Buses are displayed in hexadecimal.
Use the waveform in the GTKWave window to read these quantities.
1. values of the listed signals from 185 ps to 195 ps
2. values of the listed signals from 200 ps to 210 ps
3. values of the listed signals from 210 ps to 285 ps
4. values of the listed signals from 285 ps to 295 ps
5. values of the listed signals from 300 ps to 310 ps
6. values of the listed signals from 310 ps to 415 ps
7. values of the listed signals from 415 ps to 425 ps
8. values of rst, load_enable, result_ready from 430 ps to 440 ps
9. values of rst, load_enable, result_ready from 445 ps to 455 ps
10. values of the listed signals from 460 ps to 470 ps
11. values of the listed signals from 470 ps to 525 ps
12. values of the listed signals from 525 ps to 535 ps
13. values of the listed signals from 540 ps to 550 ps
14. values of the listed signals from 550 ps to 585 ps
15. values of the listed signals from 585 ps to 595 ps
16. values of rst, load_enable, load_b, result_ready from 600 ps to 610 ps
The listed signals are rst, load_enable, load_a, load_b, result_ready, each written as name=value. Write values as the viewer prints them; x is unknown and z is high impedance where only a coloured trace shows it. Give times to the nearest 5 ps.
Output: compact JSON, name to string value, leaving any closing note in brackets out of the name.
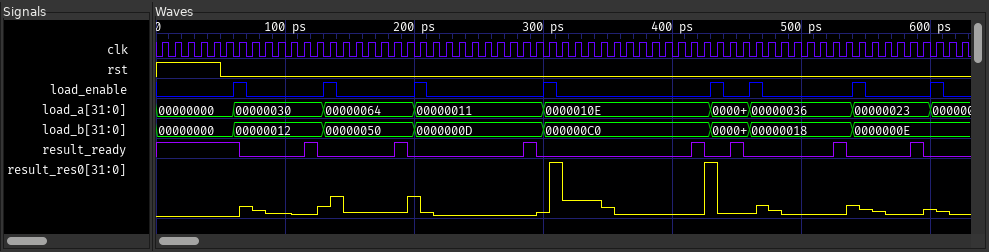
{"values of the listed signals from 185 ps to 195 ps": "rst=0, load_enable=0, load_a=00000064, load_b=00000050, result_ready=1", "values of the listed signals from 200 ps to 210 ps": "rst=0, load_enable=1, load_a=00000011, load_b=0000000D, result_ready=0", "values of the listed signals from 210 ps to 285 ps": "rst=0, load_enable=0, load_a=00000011, load_b=0000000D, result_ready=0", "values of the listed signals from 285 ps to 295 ps": "rst=0, load_enable=0, load_a=00000011, load_b=0000000D, result_ready=1", "values of the listed signals from 300 ps to 310 ps": "rst=0, load_enable=1, load_a=0000010E, load_b=000000C0, result_ready=0", "values of the listed signals from 310 ps to 415 ps": "rst=0, load_enable=0, load_a=0000010E, load_b=000000C0, result_ready=0", "values of the listed signals from 415 ps to 425 ps": "rst=0, load_enable=0, load_a=0000010E, load_b=000000C0, result_ready=1", "values of rst, load_enable, result_ready from 430 ps to 440 ps": "rst=0, load_enable=1, result_ready=0", "values of rst, load_enable, result_ready from 445 ps to 455 ps": "rst=0, load_enable=0, result_ready=1", "values of the listed signals from 460 ps to 470 ps": "rst=0, load_enable=1, load_a=00000036, load_b=00000018, result_ready=0", "values of the listed signals from 470 ps to 525 ps": "rst=0, load_enable=0, load_a=00000036, load_b=00000018, result_ready=0", "values of the listed signals from 525 ps to 535 ps": "rst=0, load_enable=0, load_a=00000036, load_b=00000018, result_ready=1", "values of the listed signals from 540 ps to 550 ps": "rst=0, load_enable=1, load_a=00000023, load_b=0000000E, result_ready=0", "values of the listed signals from 550 ps to 585 ps": "rst=0, load_enable=0, load_a=00000023, load_b=0000000E, result_ready=0", "values of the listed signals from 585 ps to 595 ps": "rst=0, load_enable=0, load_a=00000023, load_b=0000000E, result_ready=1", "values of rst, load_enable, load_b, result_ready from 600 ps to 610 ps": "rst=0, load_enable=1, load_b=0000000E, result_ready=0"}
